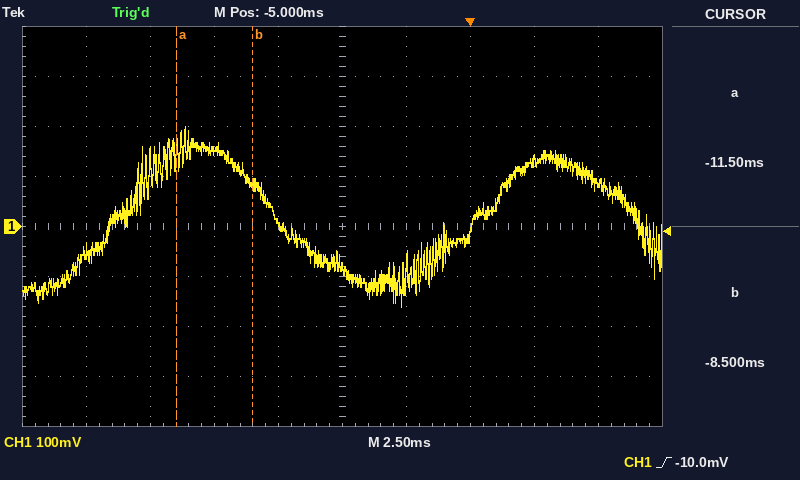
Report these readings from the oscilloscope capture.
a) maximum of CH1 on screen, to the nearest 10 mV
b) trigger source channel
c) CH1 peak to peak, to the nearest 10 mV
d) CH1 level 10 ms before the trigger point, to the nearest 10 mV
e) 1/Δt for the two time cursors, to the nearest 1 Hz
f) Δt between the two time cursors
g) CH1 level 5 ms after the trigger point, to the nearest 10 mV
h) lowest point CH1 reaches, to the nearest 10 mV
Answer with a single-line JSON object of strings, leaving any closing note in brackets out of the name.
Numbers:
{"maximum of CH1 on screen, to the nearest 10 mV": "200 mV", "trigger source channel": "CH1", "CH1 peak to peak, to the nearest 10 mV": "360 mV", "CH1 level 10 ms before the trigger point, to the nearest 10 mV": "150 mV", "1/Δt for the two time cursors, to the nearest 1 Hz": "333 Hz", "Δt between the two time cursors": "3.00 ms", "CH1 level 5 ms after the trigger point, to the nearest 10 mV": "90 mV", "lowest point CH1 reaches, to the nearest 10 mV": "-160 mV"}
